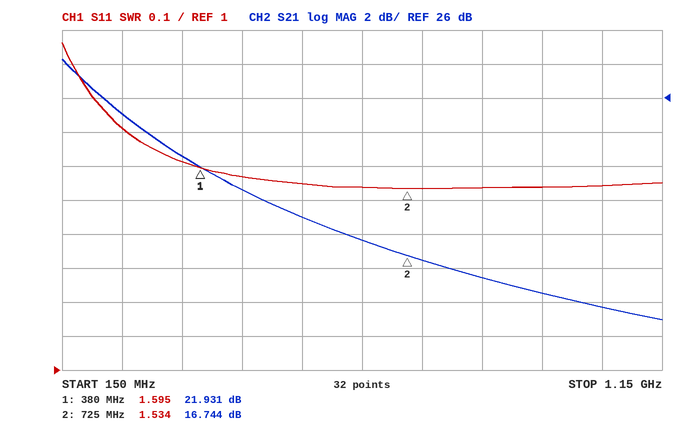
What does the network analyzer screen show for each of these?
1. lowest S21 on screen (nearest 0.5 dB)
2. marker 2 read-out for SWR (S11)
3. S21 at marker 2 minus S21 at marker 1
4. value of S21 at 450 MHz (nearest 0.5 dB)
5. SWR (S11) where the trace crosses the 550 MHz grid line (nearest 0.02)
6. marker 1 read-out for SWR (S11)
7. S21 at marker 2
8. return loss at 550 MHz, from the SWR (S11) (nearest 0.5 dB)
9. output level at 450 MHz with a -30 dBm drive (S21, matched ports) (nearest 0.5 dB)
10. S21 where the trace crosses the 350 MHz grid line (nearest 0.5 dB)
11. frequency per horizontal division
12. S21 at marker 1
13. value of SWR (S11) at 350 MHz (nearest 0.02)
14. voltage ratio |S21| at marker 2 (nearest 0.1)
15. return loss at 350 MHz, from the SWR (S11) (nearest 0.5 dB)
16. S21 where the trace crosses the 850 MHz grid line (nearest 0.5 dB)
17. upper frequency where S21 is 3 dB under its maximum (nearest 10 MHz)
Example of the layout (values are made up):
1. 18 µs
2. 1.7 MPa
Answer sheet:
1. 13.0 dB
2. 1.534
3. -5.187 dB
4. 20.5 dB
5. 1.54
6. 1.595
7. 16.744 dB
8. 13.5 dB
9. -9.5 dBm
10. 22.5 dB
11. 100 MHz
12. 21.931 dB
13. 1.62
14. 6.9
15. 12.5 dB
16. 15.5 dB
17. 240 MHz
